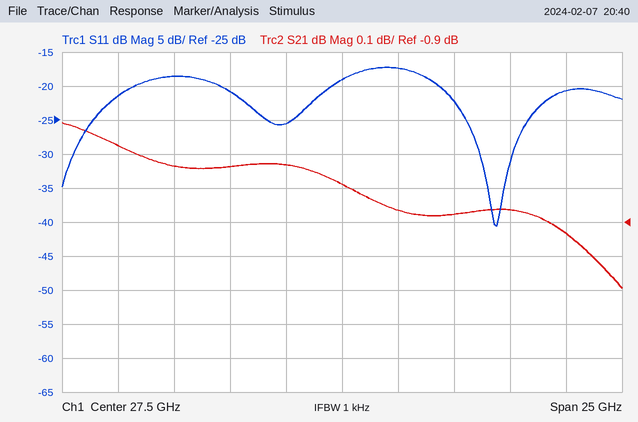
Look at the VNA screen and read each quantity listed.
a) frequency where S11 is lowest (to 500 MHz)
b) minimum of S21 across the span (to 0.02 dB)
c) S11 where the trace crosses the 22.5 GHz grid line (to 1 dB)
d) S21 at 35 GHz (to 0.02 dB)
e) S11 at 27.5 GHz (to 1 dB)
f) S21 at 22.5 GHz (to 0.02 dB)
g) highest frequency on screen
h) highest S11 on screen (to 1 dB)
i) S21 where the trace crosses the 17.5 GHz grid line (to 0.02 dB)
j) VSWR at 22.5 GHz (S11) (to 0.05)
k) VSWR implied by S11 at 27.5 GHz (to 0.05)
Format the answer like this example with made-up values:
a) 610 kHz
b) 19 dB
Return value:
a) 34.5 GHz
b) -1.10 dB
c) -21 dB
d) -0.86 dB
e) -19 dB
f) -0.74 dB
g) 40 GHz
h) -17 dB
i) -0.68 dB
j) 1.20
k) 1.25
